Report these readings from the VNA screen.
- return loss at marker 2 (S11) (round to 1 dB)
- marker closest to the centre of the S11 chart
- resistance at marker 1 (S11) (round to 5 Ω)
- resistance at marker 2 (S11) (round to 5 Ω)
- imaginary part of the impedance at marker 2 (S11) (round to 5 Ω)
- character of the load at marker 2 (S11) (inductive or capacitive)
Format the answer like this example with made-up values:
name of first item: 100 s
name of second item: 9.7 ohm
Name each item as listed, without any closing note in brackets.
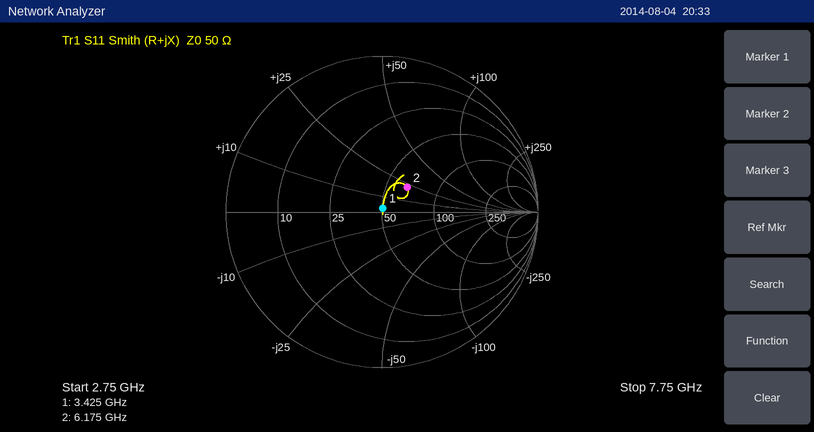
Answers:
return loss at marker 2 (S11): 13 dB
marker closest to the centre of the S11 chart: marker 1
resistance at marker 1 (S11): 50 Ω
resistance at marker 2 (S11): 65 Ω
imaginary part of the impedance at marker 2 (S11): +20 Ω
character of the load at marker 2 (S11): inductive
